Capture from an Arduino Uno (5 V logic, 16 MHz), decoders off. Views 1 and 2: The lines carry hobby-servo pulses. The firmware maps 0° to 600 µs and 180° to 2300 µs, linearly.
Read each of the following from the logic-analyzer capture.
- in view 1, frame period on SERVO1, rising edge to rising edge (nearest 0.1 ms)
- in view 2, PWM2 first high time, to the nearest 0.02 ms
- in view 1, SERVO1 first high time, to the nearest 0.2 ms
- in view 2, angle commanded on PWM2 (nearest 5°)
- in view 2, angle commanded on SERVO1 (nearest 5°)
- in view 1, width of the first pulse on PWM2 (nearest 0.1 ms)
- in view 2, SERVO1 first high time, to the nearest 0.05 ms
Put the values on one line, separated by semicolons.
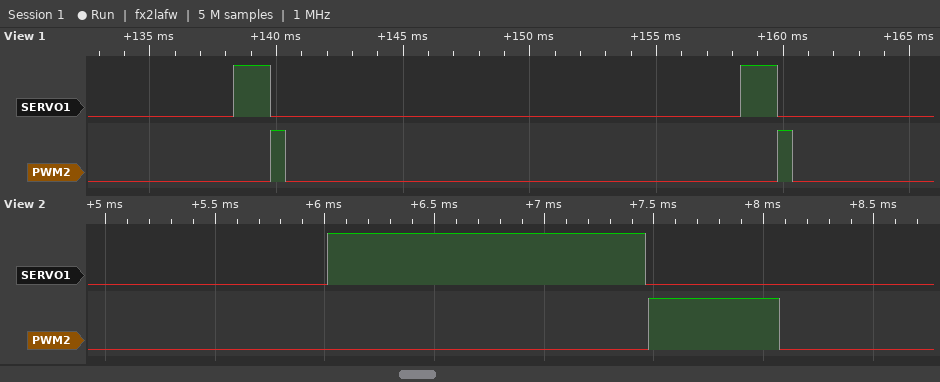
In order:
20.0 ms; 0.60 ms; 1.4 ms; 0°; 90°; 0.6 ms; 1.45 ms
